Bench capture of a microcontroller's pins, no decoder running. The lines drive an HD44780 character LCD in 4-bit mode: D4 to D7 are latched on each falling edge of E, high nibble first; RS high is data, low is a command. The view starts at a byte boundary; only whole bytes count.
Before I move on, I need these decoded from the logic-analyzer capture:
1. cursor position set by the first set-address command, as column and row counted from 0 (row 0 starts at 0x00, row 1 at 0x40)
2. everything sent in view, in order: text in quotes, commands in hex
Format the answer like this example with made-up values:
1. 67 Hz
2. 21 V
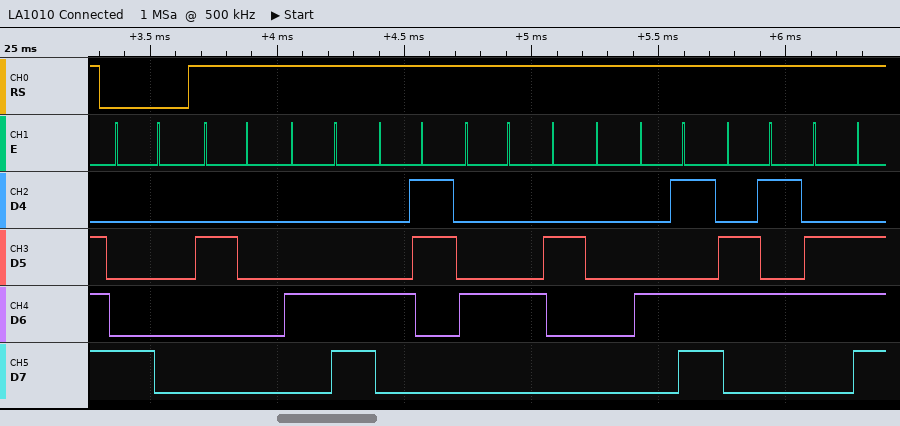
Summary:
1. column 0, row 0
2. 0x80 " LCD Men"
